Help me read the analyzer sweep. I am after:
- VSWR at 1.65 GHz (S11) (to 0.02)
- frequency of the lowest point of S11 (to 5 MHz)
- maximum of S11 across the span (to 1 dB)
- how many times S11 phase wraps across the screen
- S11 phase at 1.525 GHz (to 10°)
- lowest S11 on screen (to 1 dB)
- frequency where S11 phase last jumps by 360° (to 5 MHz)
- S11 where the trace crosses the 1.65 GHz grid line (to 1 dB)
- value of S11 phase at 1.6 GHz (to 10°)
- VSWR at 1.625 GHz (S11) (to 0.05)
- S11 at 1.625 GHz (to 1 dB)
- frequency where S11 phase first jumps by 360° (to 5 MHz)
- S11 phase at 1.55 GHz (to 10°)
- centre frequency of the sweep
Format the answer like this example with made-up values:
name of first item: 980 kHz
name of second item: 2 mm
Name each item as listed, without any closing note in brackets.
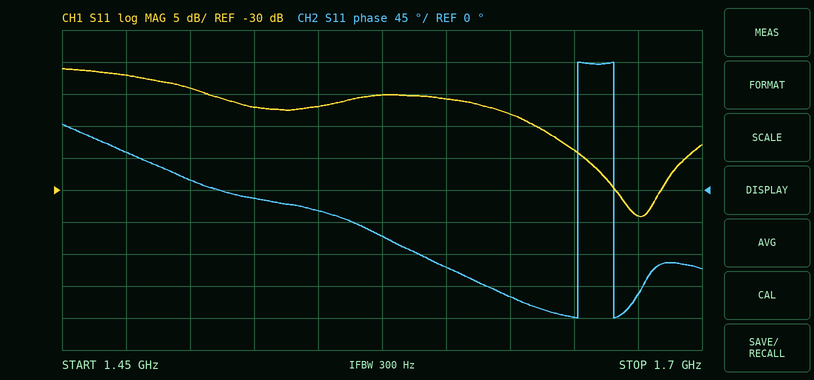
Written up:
VSWR at 1.65 GHz (S11): 1.14
frequency of the lowest point of S11: 1.675 GHz
maximum of S11 across the span: -11 dB
how many times S11 phase wraps across the screen: 2
S11 phase at 1.525 GHz: -10°
lowest S11 on screen: -34 dB
frequency where S11 phase last jumps by 360°: 1.665 GHz
S11 where the trace crosses the 1.65 GHz grid line: -24 dB
value of S11 phase at 1.6 GHz: -110°
VSWR at 1.625 GHz (S11): 1.30
S11 at 1.625 GHz: -18 dB
frequency where S11 phase first jumps by 360°: 1.650 GHz
S11 phase at 1.55 GHz: -30°
centre frequency of the sweep: 1.575 GHz
